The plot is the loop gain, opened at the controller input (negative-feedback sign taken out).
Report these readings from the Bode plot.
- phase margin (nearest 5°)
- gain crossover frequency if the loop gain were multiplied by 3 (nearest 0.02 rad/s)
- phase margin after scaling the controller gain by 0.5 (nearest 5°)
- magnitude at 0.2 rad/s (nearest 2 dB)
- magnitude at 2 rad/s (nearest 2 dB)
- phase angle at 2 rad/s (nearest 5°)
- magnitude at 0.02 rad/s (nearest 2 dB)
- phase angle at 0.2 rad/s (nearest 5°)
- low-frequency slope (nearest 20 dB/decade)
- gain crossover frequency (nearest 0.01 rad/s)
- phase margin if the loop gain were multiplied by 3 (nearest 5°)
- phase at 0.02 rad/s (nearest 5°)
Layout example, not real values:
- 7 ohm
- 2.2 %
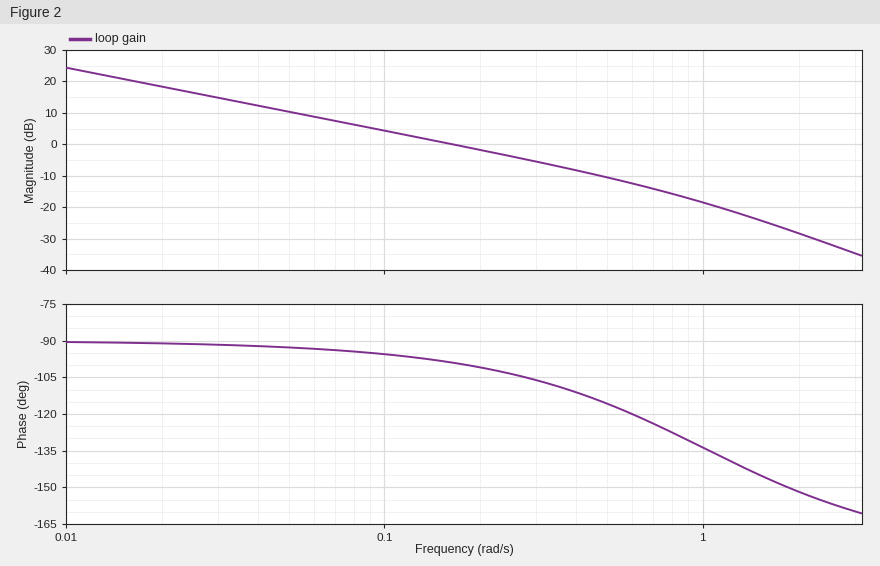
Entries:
- 80°
- 0.46 rad/s
- 85°
- -2 dB
- -28 dB
- -150°
- 18 dB
- -100°
- -20 dB/decade
- 0.16 rad/s
- 65°
- -90°
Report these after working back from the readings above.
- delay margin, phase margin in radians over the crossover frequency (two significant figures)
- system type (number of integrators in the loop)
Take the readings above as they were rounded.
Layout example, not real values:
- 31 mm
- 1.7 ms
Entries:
- 8.7 s
- 1
